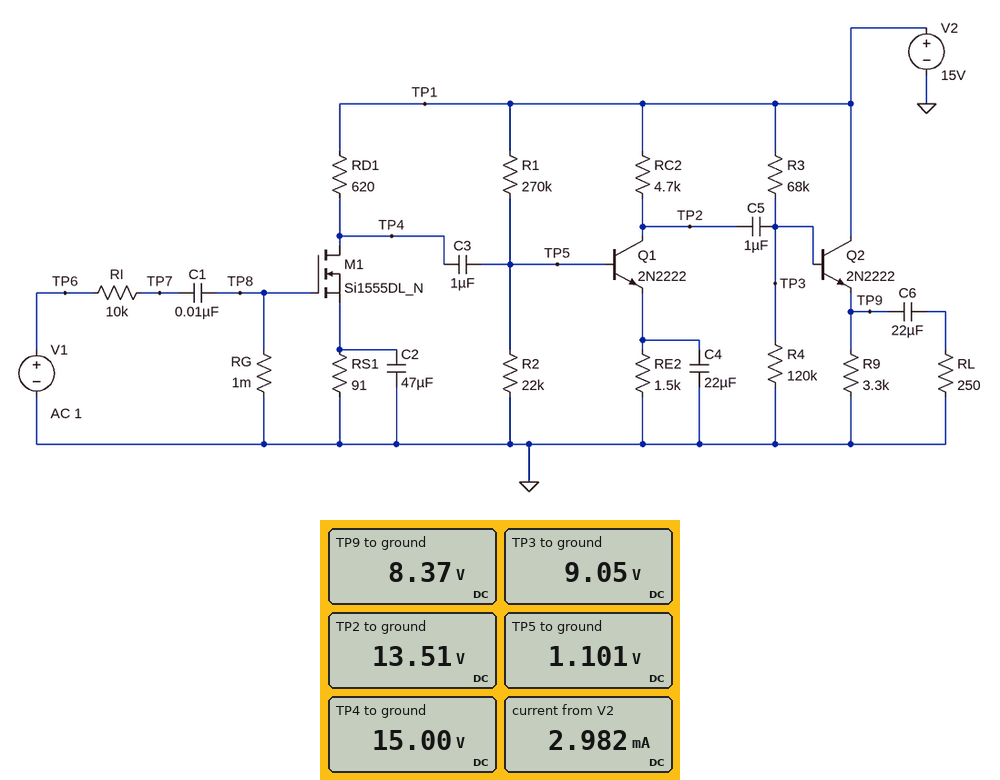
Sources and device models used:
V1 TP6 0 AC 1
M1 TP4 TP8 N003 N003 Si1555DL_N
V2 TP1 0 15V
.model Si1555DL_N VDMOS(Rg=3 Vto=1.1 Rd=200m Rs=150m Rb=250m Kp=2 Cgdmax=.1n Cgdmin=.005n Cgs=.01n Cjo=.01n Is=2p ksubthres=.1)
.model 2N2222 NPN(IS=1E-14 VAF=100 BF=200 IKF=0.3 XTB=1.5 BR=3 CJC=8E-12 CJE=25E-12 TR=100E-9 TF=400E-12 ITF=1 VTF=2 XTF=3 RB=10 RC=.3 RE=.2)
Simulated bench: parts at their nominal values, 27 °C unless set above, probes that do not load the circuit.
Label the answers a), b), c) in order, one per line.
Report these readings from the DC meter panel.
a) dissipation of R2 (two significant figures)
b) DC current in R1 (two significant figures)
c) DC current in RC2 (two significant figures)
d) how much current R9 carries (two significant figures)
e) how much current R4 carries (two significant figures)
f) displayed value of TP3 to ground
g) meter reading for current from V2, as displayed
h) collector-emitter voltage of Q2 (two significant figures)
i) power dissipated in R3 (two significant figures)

a) 55 µW
b) 51 µA
c) 320 µA
d) 2.5 mA
e) 75 µA
f) 9.05 V
g) 2.982 mA
h) 6.6 V
i) 520 µW
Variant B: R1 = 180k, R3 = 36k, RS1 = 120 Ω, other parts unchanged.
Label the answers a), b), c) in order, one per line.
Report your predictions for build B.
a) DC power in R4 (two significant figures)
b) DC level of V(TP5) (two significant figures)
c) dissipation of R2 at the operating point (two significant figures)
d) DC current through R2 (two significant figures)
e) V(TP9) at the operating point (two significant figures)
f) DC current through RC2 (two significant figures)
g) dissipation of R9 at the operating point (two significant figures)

a) 1.0 mW
b) 1.6 V
c) 110 µW
d) 72 µA
e) 10 V
f) 620 µA
g) 33 mW
